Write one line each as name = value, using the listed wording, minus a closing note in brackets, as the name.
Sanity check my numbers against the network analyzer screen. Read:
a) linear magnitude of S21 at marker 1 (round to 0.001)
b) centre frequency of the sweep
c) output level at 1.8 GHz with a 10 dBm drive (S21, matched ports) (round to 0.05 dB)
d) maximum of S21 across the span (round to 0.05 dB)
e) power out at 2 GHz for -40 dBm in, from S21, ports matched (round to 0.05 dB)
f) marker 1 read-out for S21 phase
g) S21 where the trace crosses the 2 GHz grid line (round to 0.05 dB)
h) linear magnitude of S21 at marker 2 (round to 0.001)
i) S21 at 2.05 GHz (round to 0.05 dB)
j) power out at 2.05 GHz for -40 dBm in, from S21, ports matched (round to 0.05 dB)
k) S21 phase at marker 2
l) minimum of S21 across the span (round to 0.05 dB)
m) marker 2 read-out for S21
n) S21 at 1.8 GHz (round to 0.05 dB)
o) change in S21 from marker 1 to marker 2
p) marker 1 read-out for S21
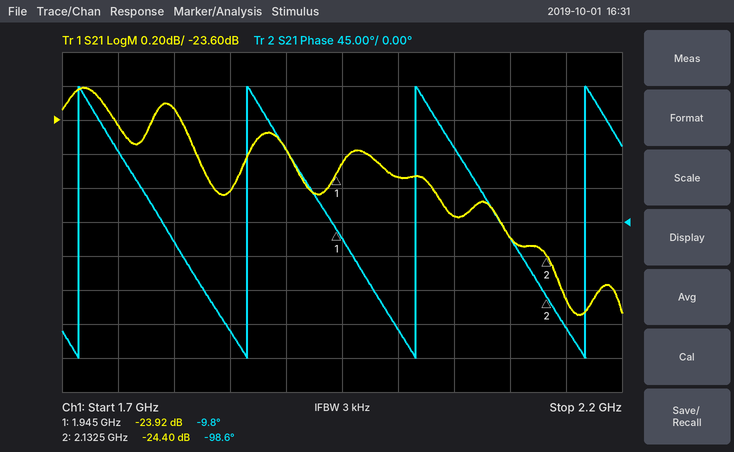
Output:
linear magnitude of S21 at marker 1 = 0.064
centre frequency of the sweep = 1.95 GHz
output level at 1.8 GHz with a 10 dBm drive (S21, matched ports) = -13.55 dBm
maximum of S21 across the span = -23.40 dB
power out at 2 GHz for -40 dBm in, from S21, ports matched = -63.95 dBm
marker 1 read-out for S21 phase = -9.8°
S21 where the trace crosses the 2 GHz grid line = -23.95 dB
linear magnitude of S21 at marker 2 = 0.060
S21 at 2.05 GHz = -24.15 dB
power out at 2.05 GHz for -40 dBm in, from S21, ports matched = -64.15 dBm
S21 phase at marker 2 = -98.6°
minimum of S21 across the span = -24.75 dB
marker 2 read-out for S21 = -24.40 dB
S21 at 1.8 GHz = -23.55 dB
change in S21 from marker 1 to marker 2 = -0.48 dB
marker 1 read-out for S21 = -23.92 dB
